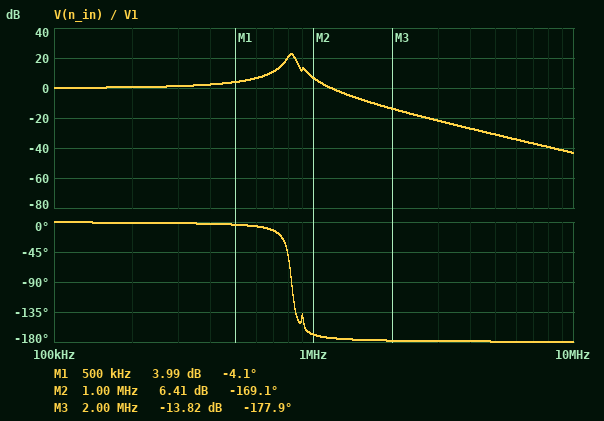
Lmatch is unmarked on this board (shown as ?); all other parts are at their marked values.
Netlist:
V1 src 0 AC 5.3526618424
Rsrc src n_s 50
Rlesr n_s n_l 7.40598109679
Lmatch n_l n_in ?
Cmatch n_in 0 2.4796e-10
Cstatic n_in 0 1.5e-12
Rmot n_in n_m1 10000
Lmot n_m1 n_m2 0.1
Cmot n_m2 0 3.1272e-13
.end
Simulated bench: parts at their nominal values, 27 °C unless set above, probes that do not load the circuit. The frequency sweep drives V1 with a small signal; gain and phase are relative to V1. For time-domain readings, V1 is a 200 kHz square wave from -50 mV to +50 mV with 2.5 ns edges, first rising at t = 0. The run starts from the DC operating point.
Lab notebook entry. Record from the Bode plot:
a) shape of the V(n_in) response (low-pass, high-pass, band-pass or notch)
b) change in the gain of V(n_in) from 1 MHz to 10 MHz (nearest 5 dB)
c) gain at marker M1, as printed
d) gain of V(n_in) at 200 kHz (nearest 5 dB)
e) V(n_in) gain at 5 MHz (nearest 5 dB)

low-pass
-50 dB
3.99 dB
0 dB
-30 dB
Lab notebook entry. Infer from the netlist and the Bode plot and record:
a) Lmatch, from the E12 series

150 µH
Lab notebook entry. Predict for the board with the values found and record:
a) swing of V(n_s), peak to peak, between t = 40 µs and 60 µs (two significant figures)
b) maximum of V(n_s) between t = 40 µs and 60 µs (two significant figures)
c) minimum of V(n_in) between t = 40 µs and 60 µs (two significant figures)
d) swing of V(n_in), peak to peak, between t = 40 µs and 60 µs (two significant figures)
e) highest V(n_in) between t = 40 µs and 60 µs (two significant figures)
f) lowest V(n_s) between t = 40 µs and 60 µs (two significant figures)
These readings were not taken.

110 mV
53 mV
-110 mV
210 mV
110 mV
-53 mV
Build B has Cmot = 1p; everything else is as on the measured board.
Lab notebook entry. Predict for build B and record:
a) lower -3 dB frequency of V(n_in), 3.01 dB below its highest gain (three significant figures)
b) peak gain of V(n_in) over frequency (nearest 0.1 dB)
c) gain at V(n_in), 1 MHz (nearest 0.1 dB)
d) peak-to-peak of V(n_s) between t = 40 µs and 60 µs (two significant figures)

792 kHz
22.6 dB
6.3 dB
110 mV
